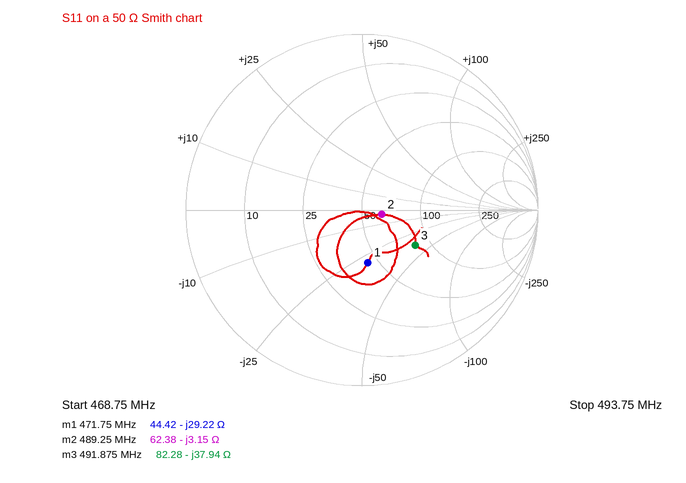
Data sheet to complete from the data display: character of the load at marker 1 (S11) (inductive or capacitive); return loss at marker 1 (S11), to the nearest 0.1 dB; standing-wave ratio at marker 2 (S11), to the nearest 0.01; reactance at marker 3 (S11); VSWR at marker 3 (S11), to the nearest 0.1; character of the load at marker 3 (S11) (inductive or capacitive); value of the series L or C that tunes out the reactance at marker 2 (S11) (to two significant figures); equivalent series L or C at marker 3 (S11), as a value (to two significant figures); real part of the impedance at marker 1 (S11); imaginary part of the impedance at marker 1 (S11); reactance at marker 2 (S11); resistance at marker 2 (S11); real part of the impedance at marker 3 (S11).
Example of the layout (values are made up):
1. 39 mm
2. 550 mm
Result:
1. capacitive
2. 10.4 dB
3. 1.26
4. -37.94 Ω
5. 2.1
6. capacitive
7. 1.0 nH
8. 8.5 pF
9. 44.42 Ω
10. -29.22 Ω
11. -3.15 Ω
12. 62.38 Ω
13. 82.28 Ω
